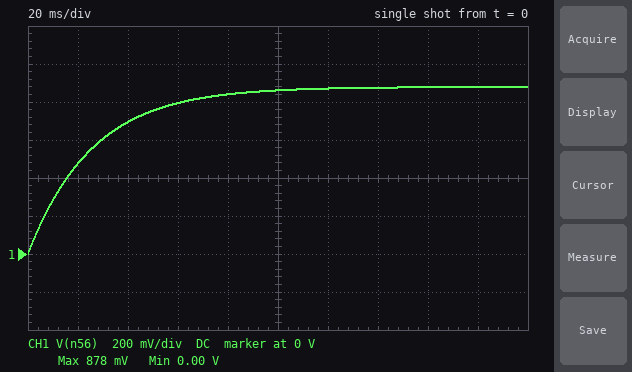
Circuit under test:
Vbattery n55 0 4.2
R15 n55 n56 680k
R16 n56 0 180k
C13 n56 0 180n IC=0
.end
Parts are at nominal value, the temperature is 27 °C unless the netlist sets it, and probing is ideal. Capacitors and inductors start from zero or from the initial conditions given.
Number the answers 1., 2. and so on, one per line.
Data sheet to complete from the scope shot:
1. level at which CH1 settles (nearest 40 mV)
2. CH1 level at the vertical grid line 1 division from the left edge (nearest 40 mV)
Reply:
1. 880 mV
2. 480 mV
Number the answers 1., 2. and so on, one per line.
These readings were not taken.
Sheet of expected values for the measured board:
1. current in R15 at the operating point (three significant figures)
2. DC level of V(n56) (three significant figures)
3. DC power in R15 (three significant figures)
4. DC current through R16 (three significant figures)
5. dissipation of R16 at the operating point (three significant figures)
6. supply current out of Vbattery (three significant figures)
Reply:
1. 4.88 µA
2. 879 mV
3. 16.2 µW
4. 4.88 µA
5. 4.29 µW
6. 4.88 µA
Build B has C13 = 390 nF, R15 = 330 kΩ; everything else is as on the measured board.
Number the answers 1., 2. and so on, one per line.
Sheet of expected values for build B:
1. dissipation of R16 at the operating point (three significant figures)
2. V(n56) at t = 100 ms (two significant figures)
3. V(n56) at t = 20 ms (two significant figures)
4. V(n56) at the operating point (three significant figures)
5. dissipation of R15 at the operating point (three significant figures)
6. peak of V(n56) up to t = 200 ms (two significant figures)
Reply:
1. 12.2 µW
2. 1.3 V
3. 530 mV
4. 1.48 V
5. 22.4 µW
6. 1.5 V
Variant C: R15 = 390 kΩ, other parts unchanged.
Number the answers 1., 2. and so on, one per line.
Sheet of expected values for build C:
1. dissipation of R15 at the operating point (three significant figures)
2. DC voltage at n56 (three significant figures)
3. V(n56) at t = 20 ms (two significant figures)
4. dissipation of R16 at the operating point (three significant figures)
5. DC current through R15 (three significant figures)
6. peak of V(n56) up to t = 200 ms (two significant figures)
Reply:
1. 21.2 µW
2. 1.33 V
3. 790 mV
4. 9.77 µW
5. 7.37 µA
6. 1.3 V
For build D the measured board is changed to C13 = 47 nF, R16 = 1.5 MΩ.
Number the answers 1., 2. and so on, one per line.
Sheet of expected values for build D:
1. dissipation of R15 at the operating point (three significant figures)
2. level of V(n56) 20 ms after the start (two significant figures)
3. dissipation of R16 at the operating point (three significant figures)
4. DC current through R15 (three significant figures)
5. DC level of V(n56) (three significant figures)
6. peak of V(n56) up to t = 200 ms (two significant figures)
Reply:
1. 2.52 µW
2. 1.7 V
3. 5.57 µW
4. 1.93 µA
5. 2.89 V
6. 2.9 V
